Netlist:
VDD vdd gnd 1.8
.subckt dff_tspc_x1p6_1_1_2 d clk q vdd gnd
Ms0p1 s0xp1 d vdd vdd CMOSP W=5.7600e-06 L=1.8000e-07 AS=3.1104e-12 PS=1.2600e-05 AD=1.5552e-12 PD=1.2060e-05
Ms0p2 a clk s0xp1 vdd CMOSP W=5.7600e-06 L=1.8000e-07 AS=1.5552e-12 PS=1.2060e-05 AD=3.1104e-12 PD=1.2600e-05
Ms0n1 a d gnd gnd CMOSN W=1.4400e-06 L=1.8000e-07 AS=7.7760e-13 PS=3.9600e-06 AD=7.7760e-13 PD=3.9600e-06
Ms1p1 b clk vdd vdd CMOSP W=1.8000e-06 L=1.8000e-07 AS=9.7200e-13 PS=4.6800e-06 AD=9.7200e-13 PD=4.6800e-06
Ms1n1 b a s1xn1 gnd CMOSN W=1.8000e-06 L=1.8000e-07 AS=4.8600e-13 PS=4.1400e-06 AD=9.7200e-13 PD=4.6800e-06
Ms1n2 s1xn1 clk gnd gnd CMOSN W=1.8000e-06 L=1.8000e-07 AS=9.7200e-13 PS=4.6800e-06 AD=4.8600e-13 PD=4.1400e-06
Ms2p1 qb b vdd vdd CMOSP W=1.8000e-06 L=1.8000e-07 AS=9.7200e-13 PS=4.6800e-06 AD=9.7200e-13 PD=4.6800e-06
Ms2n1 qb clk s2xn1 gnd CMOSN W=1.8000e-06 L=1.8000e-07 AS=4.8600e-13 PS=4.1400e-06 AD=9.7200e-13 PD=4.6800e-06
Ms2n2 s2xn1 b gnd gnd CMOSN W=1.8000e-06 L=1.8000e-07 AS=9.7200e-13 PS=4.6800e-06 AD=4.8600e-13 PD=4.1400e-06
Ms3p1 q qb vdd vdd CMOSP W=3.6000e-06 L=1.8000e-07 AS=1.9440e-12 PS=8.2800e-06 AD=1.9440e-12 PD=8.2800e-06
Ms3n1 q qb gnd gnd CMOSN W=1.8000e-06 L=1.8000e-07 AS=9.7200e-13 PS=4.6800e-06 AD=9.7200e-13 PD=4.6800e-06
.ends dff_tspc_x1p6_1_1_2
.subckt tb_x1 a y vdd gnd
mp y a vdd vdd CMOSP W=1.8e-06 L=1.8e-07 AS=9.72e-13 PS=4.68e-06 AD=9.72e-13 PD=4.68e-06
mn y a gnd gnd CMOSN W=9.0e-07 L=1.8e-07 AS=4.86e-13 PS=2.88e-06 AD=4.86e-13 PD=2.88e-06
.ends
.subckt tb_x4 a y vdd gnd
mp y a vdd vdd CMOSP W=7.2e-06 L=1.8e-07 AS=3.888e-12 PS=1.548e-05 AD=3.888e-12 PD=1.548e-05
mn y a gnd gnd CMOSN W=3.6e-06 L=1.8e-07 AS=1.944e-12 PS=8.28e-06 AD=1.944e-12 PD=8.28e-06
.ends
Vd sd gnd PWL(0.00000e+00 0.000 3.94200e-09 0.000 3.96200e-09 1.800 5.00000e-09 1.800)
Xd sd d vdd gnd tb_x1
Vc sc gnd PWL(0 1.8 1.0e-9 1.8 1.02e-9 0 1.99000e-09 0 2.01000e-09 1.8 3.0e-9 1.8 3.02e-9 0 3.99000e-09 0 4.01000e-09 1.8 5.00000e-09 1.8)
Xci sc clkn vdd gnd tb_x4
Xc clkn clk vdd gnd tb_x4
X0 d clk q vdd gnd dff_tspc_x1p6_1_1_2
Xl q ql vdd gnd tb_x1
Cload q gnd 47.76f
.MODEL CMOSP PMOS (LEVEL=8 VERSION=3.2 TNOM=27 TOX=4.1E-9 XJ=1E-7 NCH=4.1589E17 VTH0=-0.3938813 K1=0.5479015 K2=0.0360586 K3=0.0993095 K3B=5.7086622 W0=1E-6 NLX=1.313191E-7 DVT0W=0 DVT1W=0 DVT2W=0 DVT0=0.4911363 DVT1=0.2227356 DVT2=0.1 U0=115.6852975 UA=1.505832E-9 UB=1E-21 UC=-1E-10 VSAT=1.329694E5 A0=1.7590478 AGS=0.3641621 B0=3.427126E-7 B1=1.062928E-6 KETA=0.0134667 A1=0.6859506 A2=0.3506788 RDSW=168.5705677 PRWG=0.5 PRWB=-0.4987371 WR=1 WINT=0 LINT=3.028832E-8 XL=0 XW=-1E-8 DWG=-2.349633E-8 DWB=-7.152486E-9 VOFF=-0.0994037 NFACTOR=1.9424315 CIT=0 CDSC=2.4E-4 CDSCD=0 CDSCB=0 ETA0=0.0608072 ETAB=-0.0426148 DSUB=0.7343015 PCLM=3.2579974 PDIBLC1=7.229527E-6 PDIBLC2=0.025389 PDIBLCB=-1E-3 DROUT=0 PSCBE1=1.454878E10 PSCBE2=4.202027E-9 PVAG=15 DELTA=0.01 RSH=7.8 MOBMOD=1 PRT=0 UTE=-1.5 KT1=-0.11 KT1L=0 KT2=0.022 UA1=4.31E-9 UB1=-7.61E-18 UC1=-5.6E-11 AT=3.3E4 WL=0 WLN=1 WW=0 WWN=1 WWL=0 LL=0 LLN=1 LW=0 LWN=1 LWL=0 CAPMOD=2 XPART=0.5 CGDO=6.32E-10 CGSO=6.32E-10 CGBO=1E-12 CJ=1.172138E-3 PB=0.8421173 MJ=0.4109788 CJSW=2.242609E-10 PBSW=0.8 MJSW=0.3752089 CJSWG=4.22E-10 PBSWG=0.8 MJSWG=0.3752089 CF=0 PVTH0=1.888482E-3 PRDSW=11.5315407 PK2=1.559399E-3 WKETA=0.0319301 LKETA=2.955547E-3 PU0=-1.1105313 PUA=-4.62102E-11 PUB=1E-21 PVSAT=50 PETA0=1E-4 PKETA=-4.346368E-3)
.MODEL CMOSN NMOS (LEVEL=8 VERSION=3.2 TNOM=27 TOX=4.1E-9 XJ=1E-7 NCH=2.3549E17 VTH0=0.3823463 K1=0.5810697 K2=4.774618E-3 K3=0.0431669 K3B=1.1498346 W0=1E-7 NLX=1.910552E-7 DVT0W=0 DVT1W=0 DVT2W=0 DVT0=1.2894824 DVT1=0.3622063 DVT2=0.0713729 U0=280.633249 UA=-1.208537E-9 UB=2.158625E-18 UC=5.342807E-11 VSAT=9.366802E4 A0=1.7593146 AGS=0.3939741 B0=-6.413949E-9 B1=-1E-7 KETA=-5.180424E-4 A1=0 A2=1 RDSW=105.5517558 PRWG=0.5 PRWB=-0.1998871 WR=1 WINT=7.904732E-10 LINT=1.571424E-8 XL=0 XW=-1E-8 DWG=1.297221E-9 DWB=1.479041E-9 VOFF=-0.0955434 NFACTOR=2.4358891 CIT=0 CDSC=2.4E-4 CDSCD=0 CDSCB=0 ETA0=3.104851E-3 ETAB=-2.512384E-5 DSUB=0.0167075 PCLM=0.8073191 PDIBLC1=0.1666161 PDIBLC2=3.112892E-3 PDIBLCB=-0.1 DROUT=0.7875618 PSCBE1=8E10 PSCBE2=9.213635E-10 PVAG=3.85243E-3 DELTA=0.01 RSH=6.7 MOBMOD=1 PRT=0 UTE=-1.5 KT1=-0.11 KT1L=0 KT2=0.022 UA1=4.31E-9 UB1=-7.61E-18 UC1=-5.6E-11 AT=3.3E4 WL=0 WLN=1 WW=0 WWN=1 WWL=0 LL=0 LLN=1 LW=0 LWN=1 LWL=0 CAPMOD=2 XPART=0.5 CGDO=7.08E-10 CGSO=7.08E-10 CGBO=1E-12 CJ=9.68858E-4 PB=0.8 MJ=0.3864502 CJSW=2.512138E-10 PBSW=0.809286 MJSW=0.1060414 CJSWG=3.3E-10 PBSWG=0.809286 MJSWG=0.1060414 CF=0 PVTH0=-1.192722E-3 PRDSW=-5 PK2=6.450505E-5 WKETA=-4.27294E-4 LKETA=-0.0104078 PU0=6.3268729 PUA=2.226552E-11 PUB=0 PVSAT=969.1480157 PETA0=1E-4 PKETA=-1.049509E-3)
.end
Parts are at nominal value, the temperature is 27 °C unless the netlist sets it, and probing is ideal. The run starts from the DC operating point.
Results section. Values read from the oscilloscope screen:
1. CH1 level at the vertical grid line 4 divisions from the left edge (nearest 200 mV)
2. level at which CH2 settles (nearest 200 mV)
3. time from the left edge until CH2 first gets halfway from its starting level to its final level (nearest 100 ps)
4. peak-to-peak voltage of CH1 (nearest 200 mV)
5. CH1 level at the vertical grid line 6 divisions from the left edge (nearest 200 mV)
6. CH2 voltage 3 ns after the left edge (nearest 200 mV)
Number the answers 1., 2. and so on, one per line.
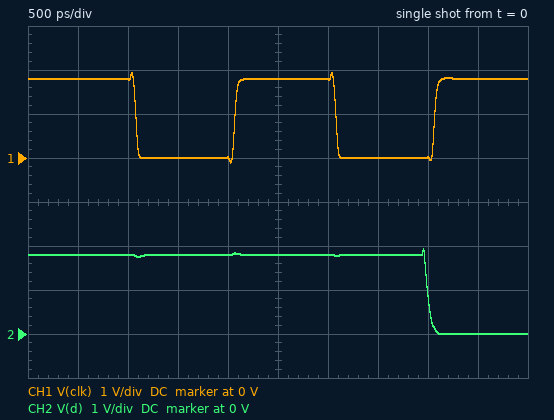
1. 0 V
2. 0 V
3. 4.0 ns
4. 2.0 V
5. 1.8 V
6. 1.8 V
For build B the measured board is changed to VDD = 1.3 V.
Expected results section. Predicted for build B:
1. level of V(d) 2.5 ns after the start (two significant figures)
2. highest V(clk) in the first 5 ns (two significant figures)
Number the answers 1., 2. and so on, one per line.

1. 1.3 V
2. 1.4 V
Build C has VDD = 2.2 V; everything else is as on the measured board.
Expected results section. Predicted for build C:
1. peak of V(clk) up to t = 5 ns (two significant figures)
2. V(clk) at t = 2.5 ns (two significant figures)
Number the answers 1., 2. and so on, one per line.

1. 2.3 V
2. 2.2 V
